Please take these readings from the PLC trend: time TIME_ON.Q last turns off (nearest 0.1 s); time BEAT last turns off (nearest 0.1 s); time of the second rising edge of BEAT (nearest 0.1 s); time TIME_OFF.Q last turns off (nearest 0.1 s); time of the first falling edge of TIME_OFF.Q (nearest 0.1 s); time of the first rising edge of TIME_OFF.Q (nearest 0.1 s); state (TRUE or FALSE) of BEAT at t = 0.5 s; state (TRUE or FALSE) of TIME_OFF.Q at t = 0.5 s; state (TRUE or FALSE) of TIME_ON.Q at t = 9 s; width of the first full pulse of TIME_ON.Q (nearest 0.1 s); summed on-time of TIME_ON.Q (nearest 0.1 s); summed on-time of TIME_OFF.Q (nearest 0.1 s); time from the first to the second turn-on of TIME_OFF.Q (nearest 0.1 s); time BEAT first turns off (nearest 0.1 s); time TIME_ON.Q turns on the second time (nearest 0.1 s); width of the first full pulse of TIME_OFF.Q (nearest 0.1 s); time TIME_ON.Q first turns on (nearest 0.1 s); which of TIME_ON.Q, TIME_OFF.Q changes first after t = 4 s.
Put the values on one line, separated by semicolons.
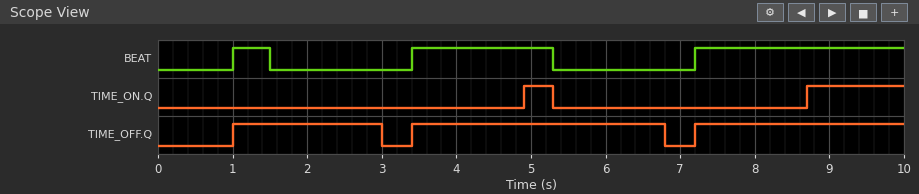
5.3 s; 5.3 s; 3.4 s; 6.8 s; 3.0 s; 1.0 s; FALSE; FALSE; TRUE; 0.4 s; 1.7 s; 8.2 s; 2.4 s; 1.5 s; 8.7 s; 2.0 s; 4.9 s; TIME_ON.Q
